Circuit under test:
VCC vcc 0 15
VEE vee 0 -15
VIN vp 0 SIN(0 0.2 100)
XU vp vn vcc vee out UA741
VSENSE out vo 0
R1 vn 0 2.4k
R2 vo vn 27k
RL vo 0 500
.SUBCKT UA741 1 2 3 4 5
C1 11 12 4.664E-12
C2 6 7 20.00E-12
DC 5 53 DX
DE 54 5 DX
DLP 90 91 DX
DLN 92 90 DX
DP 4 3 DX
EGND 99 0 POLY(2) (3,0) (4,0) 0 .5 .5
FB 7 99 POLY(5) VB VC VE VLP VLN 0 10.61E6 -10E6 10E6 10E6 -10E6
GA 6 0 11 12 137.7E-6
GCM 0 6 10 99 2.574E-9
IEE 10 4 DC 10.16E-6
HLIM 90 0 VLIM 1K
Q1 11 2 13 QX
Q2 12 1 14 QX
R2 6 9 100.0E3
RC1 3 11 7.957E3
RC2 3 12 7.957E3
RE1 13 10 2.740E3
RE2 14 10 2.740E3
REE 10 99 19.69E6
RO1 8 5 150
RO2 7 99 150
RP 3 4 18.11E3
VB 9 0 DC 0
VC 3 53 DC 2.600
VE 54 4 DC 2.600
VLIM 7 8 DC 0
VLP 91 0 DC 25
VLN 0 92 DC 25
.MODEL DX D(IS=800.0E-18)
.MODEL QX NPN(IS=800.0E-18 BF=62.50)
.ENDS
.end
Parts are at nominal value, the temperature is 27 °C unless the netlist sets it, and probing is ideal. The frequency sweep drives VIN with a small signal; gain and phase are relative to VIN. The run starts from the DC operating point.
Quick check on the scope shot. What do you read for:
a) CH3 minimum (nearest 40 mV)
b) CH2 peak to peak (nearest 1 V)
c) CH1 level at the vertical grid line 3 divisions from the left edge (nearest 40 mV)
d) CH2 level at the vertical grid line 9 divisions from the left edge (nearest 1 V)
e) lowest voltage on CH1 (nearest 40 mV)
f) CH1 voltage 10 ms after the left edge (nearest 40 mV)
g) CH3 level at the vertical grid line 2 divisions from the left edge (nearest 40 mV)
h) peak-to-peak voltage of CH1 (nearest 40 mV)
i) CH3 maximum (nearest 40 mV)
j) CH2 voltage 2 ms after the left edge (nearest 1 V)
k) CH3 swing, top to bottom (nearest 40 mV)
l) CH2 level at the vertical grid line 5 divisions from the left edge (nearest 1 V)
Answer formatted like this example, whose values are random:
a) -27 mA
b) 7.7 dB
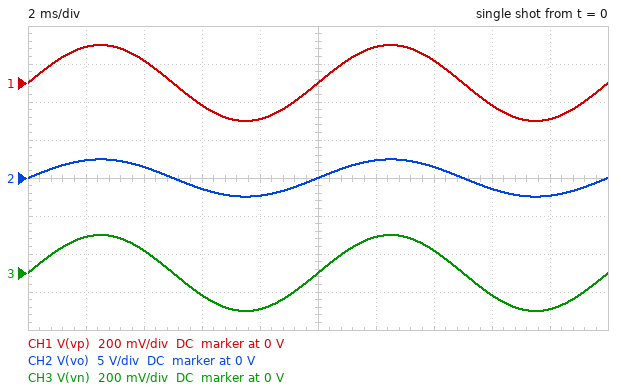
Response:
a) -200 mV
b) 5 V
c) -120 mV
d) -2 V
e) -200 mV
f) 0 V
g) 120 mV
h) 400 mV
i) 200 mV
j) 2 V
k) 400 mV
l) 0 V
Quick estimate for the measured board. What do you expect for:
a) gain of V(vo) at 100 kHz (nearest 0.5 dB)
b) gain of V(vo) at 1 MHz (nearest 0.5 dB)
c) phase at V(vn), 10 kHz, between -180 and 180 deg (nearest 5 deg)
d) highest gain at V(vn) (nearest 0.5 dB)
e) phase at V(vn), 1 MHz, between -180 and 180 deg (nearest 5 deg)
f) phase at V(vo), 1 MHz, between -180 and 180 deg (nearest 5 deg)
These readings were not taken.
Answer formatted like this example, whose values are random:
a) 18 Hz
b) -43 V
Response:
a) 17.0 dB
b) -2.0 dB
c) -10 deg
d) 0 dB
e) -110 deg
f) -110 deg
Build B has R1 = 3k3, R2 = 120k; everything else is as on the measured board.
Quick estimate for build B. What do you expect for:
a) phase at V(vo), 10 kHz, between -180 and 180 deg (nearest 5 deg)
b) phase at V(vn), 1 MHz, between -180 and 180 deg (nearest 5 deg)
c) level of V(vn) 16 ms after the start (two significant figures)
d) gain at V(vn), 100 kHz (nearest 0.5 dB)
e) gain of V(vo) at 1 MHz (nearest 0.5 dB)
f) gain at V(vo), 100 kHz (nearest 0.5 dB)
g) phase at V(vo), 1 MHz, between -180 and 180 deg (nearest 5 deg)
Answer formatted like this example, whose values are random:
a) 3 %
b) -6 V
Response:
a) -25 deg
b) -105 deg
c) -120 mV
d) -13.0 dB
e) -2.5 dB
f) 18.5 dB
g) -115 deg
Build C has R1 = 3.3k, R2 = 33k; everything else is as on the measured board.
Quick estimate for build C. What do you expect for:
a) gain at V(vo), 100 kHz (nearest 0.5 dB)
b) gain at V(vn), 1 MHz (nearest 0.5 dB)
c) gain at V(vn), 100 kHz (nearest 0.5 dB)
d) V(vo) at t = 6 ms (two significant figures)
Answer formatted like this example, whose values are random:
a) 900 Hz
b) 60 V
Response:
a) 16.5 dB
b) -23.0 dB
c) -4.0 dB
d) -1.3 V
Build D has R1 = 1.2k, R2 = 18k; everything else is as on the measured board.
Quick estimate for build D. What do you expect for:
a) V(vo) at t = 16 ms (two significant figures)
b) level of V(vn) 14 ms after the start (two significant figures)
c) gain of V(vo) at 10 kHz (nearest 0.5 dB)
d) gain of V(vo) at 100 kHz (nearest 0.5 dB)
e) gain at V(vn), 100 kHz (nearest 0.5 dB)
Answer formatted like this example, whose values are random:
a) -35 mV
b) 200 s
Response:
a) -1.9 V
b) 120 mV
c) 24.0 dB
d) 17.5 dB
e) -6.5 dB
